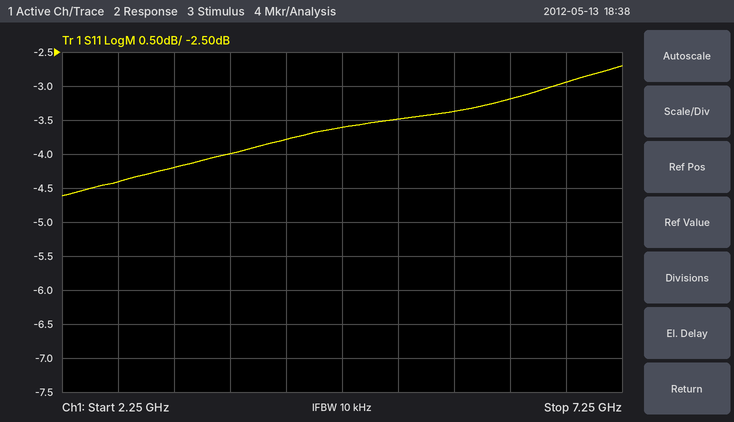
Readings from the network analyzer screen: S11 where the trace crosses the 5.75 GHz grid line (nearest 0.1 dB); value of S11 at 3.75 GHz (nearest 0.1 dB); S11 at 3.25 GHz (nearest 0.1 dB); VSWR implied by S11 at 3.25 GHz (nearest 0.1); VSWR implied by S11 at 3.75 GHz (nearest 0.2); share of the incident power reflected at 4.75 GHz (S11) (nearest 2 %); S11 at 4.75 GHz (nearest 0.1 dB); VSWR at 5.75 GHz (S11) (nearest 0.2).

-3.4 dB
-4.0 dB
-4.2 dB
4.2
4.4
44 %
-3.6 dB
5.2
